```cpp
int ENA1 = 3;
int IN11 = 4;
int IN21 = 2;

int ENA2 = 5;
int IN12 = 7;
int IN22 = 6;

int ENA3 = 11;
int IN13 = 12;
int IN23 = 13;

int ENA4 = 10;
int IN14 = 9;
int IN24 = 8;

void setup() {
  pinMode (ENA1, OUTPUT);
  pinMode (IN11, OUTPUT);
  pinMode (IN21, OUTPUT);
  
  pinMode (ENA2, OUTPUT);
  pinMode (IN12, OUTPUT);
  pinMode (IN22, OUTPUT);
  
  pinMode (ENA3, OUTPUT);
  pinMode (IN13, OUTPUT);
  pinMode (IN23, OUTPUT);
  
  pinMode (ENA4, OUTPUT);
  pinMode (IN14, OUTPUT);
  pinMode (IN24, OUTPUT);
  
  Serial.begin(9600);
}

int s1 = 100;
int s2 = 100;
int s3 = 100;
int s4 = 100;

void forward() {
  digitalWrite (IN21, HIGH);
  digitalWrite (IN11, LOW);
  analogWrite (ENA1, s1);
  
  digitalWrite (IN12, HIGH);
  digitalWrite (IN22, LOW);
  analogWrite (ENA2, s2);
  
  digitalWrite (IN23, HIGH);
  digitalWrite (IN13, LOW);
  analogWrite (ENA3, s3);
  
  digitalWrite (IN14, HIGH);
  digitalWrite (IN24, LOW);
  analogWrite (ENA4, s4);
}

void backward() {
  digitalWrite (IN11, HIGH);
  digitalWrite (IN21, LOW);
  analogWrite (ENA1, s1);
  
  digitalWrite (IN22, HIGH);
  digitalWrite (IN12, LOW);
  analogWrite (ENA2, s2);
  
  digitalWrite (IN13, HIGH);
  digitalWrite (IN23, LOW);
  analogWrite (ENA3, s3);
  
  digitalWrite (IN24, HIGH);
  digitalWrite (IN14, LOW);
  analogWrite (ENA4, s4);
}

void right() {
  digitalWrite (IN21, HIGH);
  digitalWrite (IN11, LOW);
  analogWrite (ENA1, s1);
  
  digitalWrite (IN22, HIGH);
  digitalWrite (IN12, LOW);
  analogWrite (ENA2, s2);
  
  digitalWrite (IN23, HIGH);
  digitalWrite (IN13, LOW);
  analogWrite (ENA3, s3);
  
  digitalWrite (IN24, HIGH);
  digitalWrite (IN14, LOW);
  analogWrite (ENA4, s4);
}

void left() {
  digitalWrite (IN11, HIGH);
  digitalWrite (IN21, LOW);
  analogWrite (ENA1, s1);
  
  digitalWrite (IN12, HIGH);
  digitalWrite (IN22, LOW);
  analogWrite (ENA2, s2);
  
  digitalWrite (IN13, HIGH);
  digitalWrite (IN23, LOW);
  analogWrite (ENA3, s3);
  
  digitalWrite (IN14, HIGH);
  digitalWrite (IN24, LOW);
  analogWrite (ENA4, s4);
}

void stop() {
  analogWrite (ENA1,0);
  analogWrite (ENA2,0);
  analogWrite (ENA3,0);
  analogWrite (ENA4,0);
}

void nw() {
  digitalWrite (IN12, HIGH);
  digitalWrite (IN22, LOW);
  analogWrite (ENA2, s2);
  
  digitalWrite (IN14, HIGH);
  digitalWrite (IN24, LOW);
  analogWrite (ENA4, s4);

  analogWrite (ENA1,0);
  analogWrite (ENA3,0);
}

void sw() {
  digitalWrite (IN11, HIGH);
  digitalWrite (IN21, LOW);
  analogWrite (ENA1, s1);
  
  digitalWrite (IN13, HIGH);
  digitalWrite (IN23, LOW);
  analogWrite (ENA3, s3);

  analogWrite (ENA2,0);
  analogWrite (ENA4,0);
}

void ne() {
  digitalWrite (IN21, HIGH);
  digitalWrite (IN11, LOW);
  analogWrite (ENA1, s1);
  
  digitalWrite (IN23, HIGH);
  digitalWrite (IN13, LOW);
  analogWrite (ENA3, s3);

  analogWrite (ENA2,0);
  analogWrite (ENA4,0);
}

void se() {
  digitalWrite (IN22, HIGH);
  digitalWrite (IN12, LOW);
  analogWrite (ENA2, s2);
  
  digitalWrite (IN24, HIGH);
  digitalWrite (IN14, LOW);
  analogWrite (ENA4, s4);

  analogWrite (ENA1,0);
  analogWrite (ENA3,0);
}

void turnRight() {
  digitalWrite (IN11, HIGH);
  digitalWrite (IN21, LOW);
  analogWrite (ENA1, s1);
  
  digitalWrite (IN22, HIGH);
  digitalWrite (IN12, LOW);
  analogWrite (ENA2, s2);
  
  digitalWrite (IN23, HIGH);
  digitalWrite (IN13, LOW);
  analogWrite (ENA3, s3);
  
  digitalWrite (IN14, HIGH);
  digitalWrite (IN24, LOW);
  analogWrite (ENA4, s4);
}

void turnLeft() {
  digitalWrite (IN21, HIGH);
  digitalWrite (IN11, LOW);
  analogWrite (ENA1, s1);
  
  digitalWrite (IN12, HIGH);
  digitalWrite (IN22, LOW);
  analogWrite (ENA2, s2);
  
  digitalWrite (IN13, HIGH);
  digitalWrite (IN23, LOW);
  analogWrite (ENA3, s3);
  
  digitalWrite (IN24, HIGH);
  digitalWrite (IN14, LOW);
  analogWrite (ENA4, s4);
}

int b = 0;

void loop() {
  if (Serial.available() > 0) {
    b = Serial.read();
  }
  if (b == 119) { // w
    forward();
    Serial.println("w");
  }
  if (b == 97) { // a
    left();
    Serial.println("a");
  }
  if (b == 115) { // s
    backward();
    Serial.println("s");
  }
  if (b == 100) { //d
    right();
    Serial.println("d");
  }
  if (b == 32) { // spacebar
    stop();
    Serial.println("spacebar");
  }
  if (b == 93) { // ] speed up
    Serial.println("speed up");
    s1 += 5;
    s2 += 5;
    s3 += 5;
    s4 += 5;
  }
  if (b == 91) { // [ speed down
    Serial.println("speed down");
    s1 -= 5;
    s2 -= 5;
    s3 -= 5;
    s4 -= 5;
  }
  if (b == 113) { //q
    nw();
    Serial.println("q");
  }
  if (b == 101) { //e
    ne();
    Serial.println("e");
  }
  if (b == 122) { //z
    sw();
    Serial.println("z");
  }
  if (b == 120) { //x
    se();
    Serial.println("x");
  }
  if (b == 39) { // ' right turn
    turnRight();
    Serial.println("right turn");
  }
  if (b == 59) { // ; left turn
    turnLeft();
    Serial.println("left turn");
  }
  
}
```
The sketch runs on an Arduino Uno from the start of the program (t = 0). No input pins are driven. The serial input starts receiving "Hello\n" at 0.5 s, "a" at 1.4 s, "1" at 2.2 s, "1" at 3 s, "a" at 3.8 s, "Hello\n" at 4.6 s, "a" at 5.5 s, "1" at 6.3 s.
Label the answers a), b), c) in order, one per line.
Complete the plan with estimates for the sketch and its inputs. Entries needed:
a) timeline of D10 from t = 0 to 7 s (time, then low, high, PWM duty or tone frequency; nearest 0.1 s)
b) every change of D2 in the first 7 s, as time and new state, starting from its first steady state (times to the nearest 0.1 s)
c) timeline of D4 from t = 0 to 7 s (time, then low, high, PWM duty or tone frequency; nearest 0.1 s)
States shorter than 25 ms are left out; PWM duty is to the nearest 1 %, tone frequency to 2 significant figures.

a) 0 s low; 1.4 s PWM 39 %; 4.6 s low; 5.5 s PWM 39 %
b) 0 s low; 0.5 s high; 1.4 s low; 4.6 s high; 5.5 s low
c) 0 s low; 1.4 s high; 4.6 s low; 5.5 s high
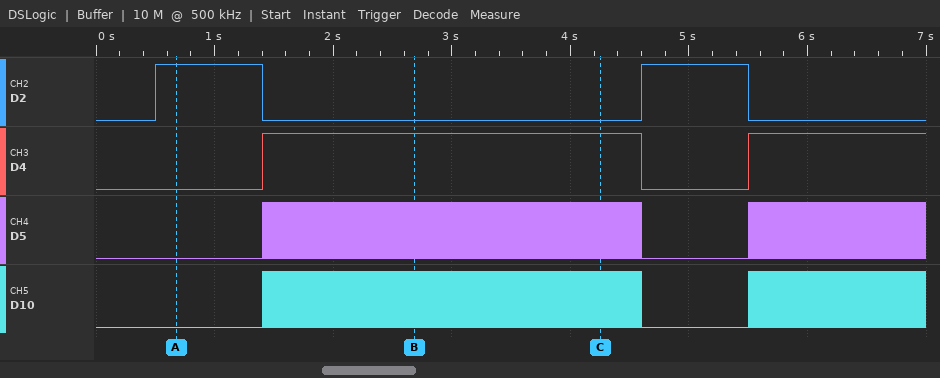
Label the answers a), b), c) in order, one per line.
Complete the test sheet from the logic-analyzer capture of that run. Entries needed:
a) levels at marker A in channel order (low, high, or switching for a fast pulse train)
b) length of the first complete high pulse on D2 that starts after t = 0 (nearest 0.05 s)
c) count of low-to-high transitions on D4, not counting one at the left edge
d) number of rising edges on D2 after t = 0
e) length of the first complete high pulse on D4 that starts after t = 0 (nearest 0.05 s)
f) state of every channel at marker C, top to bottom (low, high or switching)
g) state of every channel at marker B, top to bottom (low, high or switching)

a) D2 high, D4 low, D5 low, D10 low
b) 0.90 s
c) 2
d) 2
e) 3.20 s
f) D2 low, D4 high, D5 switching, D10 switching
g) D2 low, D4 high, D5 switching, D10 switching
